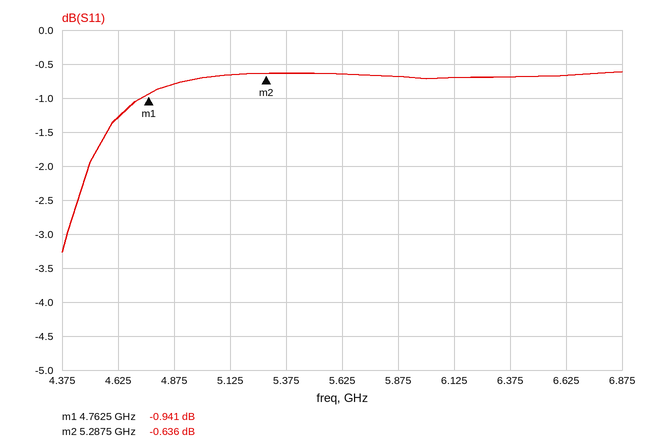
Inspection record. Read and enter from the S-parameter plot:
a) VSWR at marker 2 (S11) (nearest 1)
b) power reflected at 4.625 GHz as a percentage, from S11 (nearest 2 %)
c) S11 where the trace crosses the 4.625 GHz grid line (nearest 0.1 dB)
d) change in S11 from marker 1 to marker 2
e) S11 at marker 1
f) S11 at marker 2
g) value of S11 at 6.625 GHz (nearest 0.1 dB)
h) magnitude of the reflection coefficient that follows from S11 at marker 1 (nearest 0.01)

27
74 %
-1.3 dB
0.305 dB
-0.941 dB
-0.636 dB
-0.7 dB
0.90
